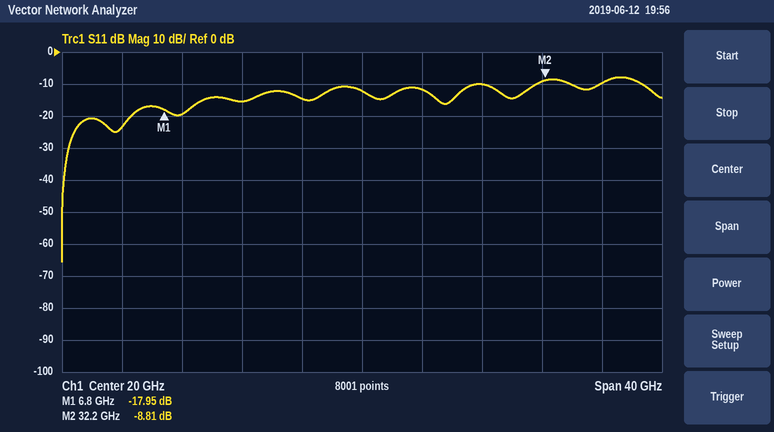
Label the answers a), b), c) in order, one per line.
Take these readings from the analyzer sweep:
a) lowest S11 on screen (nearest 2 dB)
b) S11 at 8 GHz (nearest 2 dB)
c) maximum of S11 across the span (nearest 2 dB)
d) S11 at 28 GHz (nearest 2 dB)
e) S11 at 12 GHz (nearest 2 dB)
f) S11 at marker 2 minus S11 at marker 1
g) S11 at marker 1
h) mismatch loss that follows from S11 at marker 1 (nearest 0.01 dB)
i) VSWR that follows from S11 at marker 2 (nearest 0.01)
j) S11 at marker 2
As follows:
a) -66 dB
b) -20 dB
c) -8 dB
d) -10 dB
e) -16 dB
f) 9.14 dB
g) -17.95 dB
h) 0.07 dB
i) 2.14
j) -8.81 dB
